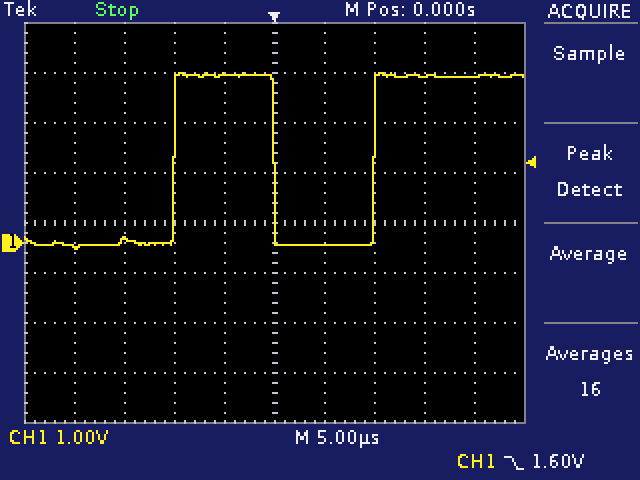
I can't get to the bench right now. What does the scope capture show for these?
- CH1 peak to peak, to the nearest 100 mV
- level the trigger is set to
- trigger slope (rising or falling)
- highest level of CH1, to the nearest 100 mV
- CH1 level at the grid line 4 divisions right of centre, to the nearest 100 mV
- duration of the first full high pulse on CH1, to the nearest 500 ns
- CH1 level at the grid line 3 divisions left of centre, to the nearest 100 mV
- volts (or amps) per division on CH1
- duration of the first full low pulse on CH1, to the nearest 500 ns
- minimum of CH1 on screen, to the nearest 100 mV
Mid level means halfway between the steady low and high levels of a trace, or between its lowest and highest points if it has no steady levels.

3.5 V
1.60 V
falling
3.4 V
3.3 V
10.0 µs
100 mV
1 V
10.0 µs
-100 mV
